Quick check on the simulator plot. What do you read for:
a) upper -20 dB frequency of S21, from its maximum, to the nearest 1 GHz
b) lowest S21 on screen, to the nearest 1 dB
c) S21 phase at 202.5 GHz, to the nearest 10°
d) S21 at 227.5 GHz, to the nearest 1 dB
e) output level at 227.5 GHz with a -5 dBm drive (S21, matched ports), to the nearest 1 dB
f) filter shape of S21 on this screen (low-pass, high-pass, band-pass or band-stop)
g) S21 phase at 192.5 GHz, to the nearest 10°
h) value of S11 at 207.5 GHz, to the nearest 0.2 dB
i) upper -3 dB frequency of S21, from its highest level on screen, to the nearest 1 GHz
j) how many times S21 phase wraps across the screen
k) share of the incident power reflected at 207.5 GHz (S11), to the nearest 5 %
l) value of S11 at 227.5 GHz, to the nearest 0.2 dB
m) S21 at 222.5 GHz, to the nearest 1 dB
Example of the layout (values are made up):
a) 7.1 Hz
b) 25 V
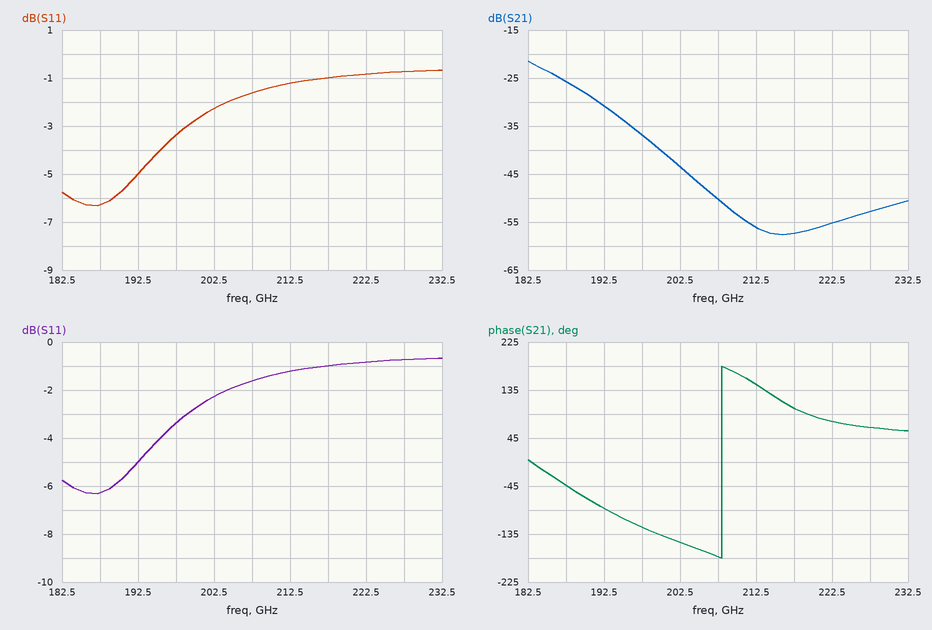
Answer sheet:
a) 201 GHz
b) -58 dB
c) -150°
d) -53 dB
e) -58 dBm
f) low-pass
g) -90°
h) -1.6 dB
i) 186 GHz
j) 1
k) 70 %
l) -0.8 dB
m) -55 dB
